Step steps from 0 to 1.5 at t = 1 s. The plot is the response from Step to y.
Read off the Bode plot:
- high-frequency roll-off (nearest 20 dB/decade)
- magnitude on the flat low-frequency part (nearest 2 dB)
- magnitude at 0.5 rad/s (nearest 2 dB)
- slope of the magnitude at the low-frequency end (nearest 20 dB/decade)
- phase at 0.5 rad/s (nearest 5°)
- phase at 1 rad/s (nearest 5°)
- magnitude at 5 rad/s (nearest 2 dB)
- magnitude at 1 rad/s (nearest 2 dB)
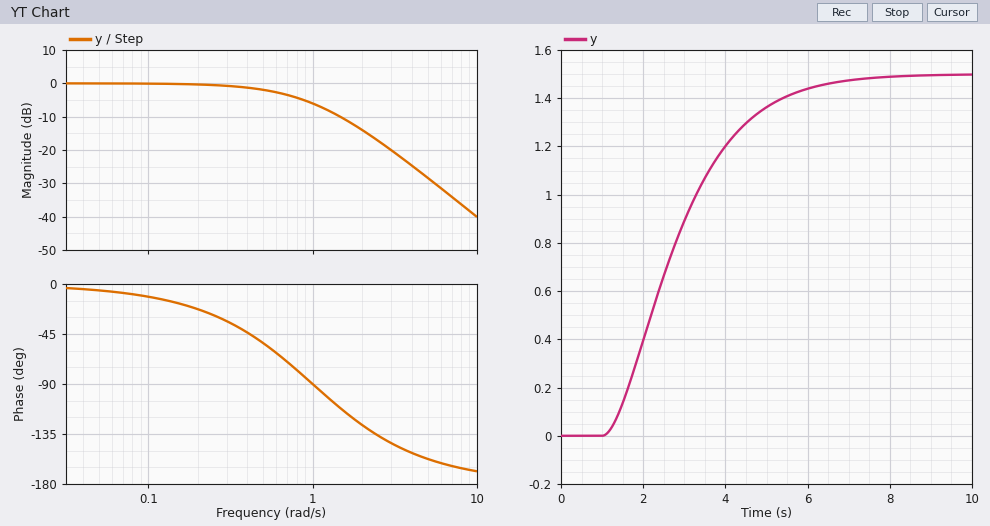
-40 dB/decade
0 dB
-2 dB
0 dB/decade
-55°
-90°
-28 dB
-6 dB
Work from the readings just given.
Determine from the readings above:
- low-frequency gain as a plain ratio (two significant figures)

1.0
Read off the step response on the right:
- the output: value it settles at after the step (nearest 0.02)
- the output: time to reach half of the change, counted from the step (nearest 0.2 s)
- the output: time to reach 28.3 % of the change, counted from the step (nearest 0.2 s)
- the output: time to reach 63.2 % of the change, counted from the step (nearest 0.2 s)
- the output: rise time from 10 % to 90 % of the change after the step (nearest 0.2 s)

1.50
1.6 s
1.0 s
2.2 s
3.4 s
